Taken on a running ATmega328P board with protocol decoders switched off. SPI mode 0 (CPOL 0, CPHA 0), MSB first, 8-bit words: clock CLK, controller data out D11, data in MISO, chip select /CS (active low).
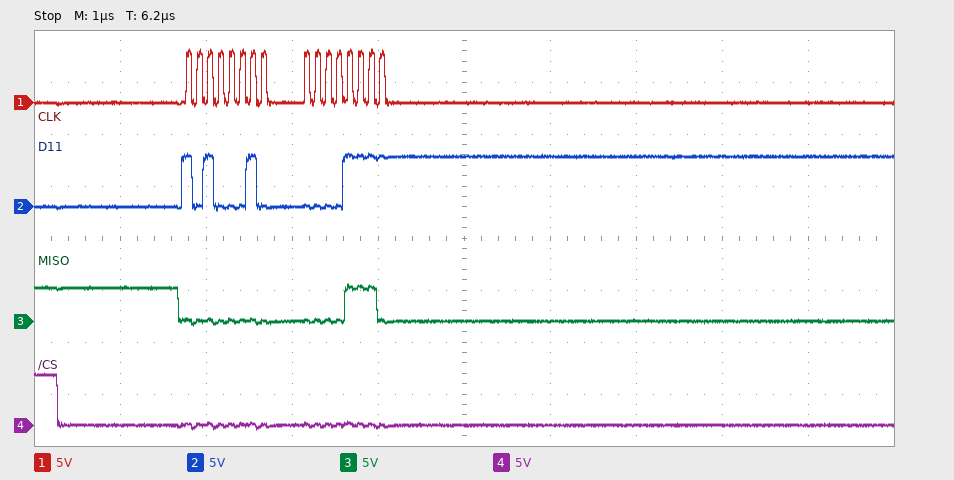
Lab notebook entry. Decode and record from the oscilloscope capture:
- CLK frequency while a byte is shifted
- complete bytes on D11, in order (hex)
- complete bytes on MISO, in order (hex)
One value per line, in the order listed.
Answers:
8 MHz
A2 0F
00 0E
